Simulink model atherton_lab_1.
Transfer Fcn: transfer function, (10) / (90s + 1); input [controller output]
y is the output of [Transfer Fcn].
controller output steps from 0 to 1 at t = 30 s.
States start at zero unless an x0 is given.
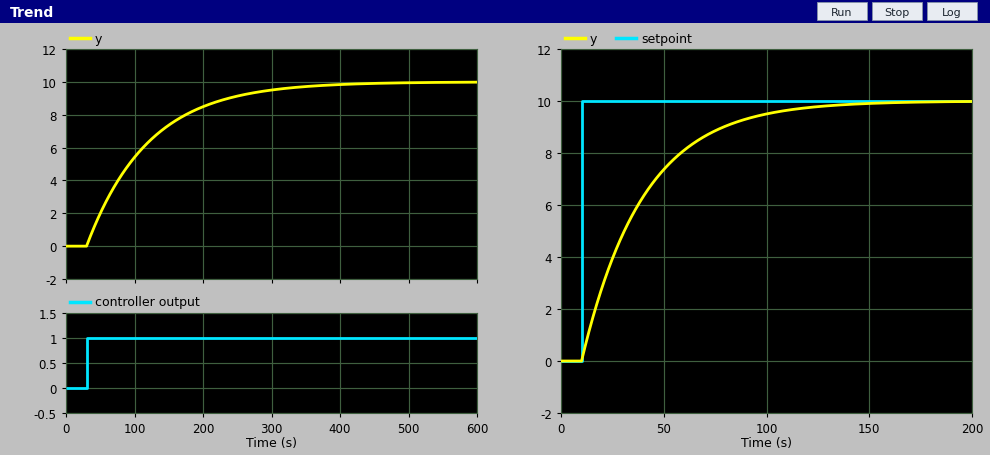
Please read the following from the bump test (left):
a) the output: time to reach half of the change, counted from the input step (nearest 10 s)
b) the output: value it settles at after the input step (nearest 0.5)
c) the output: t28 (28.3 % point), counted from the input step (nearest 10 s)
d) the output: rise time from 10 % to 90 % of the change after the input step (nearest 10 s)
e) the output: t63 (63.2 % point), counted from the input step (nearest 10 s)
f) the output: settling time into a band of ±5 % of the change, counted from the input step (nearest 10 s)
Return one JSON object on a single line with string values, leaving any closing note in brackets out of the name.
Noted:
{"the output: time to reach half of the change, counted from the input step": "60 s", "the output: value it settles at after the input step": "10.0", "the output: t28 (28.3 % point), counted from the input step": "30 s", "the output: rise time from 10 % to 90 % of the change after the input step": "200 s", "the output: t63 (63.2 % point), counted from the input step": "90 s", "the output: settling time into a band of ±5 % of the change, counted from the input step": "270 s"}
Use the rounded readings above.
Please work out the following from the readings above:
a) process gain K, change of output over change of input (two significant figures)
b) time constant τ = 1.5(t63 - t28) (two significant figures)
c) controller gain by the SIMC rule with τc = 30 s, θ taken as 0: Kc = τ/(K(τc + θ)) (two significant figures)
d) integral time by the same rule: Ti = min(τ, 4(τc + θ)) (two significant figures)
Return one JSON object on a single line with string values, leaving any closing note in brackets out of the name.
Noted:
{"process gain K, change of output over change of input": "10", "time constant τ = 1.5(t63 - t28)": "90 s", "controller gain by the SIMC rule with τc = 30 s, θ taken as 0: Kc = τ/(K(τc + θ))": "0.30", "integral time by the same rule: Ti = min(τ, 4(τc + θ))": "90 s"}
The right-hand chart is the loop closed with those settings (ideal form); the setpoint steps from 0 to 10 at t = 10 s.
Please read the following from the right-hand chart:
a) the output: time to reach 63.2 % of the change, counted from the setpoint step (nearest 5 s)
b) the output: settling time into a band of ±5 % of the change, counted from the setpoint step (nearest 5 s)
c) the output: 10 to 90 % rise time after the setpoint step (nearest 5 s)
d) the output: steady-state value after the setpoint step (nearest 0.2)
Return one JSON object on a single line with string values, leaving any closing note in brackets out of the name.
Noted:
{"the output: time to reach 63.2 % of the change, counted from the setpoint step": "30 s", "the output: settling time into a band of ±5 % of the change, counted from the setpoint step": "90 s", "the output: 10 to 90 % rise time after the setpoint step": "65 s", "the output: steady-state value after the setpoint step": "10.0"}
